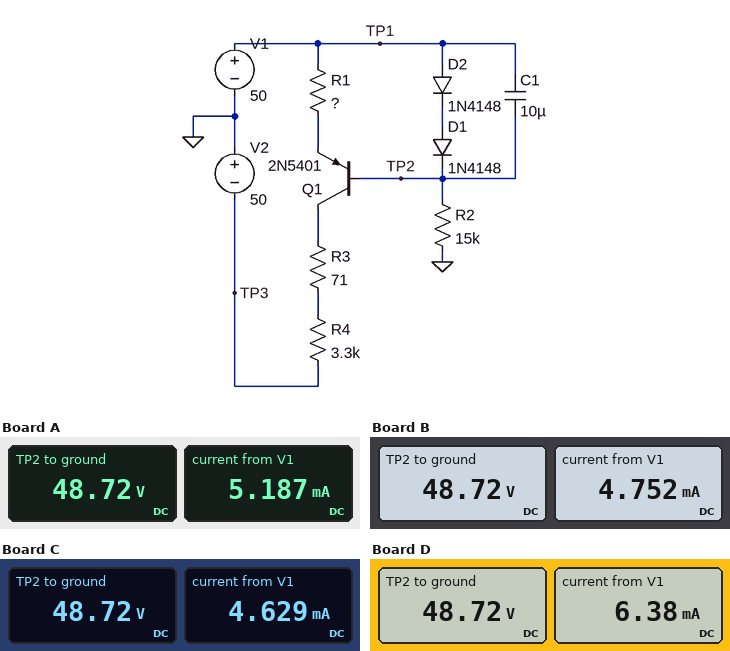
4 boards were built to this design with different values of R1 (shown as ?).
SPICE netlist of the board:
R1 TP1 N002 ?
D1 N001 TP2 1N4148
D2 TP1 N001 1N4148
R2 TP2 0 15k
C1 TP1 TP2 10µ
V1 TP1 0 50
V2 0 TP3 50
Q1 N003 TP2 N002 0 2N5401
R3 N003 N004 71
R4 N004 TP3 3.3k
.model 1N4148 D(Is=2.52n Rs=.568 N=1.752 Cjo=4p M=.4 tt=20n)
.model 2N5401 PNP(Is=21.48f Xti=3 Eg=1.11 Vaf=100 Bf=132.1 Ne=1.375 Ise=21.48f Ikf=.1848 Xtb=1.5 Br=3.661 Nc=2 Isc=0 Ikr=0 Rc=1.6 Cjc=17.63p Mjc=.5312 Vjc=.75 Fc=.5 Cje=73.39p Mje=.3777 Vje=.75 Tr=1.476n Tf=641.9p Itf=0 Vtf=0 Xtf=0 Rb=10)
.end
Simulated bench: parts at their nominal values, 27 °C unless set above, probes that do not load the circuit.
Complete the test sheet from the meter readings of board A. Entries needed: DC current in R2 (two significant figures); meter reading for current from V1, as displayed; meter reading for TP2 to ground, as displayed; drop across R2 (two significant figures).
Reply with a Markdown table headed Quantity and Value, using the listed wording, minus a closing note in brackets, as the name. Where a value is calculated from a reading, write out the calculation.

| Quantity | Value |
|---|---|
| DC current in R2 | (48.72 V) / 15 kΩ = 3.2 mA |
| meter reading for current from V1, as displayed | 5.187 mA |
| meter reading for TP2 to ground, as displayed | 48.72 V |
| drop across R2 | 48.72 V = 49 V |
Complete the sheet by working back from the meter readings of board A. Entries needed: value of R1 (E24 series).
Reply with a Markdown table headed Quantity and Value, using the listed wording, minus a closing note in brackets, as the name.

| Quantity | Value |
|---|---|
| value of R1 | 330 Ω |
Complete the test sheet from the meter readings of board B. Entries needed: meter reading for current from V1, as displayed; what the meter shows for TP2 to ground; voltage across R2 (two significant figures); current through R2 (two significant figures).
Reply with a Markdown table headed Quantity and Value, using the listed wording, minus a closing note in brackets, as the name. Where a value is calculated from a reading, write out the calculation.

| Quantity | Value |
|---|---|
| meter reading for current from V1, as displayed | 4.752 mA |
| what the meter shows for TP2 to ground | 48.72 V |
| voltage across R2 | 48.72 V = 49 V |
| current through R2 | (48.72 V) / 15 kΩ = 3.2 mA |
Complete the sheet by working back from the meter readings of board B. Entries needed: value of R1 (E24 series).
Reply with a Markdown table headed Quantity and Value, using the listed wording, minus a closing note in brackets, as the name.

| Quantity | Value |
|---|---|
| value of R1 | 430 Ω |
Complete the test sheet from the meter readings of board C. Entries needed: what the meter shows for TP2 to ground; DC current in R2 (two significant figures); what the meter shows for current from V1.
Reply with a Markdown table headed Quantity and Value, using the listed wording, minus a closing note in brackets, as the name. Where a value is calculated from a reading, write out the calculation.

| Quantity | Value |
|---|---|
| what the meter shows for TP2 to ground | 48.72 V |
| DC current in R2 | (48.72 V) / 15 kΩ = 3.2 mA |
| what the meter shows for current from V1 | 4.629 mA |
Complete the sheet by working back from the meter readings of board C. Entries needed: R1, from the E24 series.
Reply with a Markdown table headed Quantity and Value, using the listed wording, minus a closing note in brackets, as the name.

| Quantity | Value |
|---|---|
| R1, from the E24 series | 470 Ω |
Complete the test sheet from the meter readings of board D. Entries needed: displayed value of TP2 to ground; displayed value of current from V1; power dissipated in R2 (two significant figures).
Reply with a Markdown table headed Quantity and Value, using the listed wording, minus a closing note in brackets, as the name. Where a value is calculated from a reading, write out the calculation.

| Quantity | Value |
|---|---|
| displayed value of TP2 to ground | 48.72 V |
| displayed value of current from V1 | 6.38 mA |
| power dissipated in R2 | (48.72 V)^2 / 15 kΩ = 160 mW |
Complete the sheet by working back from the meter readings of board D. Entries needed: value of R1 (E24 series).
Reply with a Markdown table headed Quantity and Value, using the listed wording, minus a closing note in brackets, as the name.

| Quantity | Value |
|---|---|
| value of R1 | 200 Ω |
